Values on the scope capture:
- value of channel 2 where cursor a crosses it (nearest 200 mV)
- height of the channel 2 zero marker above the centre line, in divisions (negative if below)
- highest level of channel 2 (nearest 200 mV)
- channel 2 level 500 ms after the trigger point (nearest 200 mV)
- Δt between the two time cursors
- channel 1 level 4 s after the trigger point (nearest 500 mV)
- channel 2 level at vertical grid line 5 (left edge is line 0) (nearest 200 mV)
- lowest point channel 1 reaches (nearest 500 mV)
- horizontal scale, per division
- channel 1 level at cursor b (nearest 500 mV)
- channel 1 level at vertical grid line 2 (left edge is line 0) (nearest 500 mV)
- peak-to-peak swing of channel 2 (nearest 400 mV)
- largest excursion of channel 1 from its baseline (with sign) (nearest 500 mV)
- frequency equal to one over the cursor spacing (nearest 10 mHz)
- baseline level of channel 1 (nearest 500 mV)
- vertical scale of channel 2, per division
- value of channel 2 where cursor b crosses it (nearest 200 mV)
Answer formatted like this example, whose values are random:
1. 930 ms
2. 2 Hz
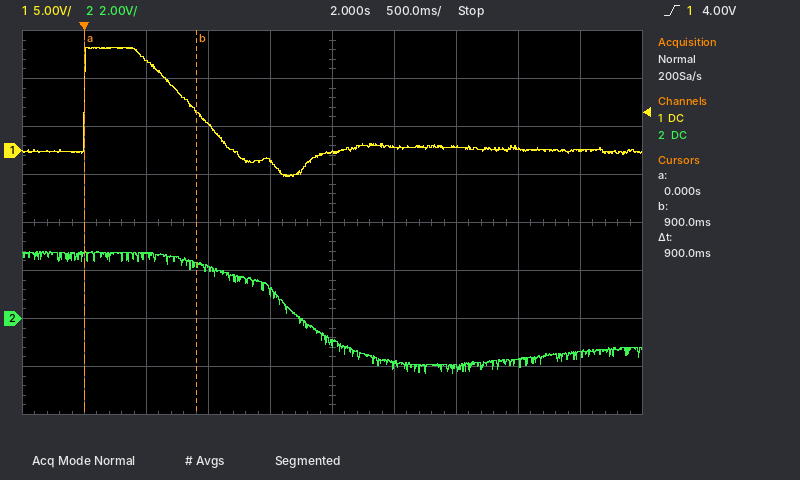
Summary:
1. 2.6 V
2. -2.0 div
3. 2.8 V
4. 2.6 V
5. 900 ms
6. 0.0 V
7. -1.0 V
8. -2.5 V
9. 500 ms
10. 4.0 V
11. 9.5 V
12. 5.2 V
13. +10.5 V
14. 1.11 Hz
15. 0.0 V
16. 2 V
17. 2.2 V
